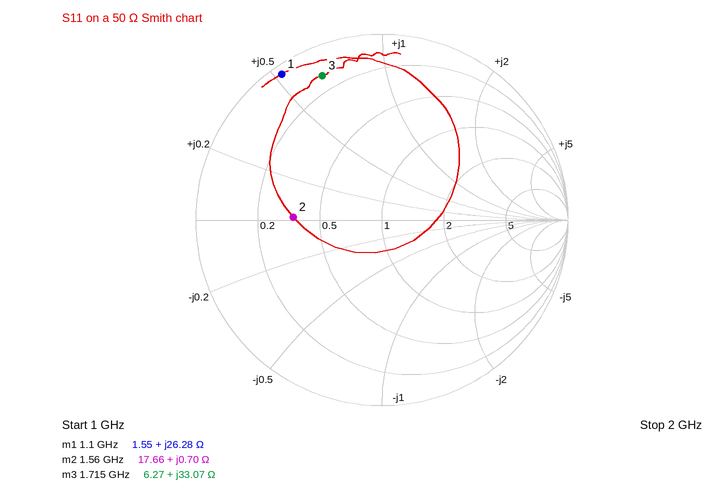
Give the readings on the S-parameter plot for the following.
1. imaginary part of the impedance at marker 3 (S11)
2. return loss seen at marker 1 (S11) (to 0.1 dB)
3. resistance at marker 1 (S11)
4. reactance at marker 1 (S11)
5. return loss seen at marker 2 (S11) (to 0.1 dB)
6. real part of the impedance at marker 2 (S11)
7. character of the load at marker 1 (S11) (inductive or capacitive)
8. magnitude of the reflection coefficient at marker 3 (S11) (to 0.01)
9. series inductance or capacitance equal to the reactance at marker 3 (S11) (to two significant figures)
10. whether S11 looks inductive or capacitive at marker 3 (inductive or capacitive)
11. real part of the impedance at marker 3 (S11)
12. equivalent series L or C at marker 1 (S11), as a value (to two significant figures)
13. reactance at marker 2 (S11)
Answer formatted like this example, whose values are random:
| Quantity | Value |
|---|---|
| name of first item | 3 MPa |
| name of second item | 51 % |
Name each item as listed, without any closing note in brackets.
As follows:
| Quantity | Value |
|---|---|
| imaginary part of the impedance at marker 3 | +33.07 Ω |
| return loss seen at marker 1 (S11) | 0.4 dB |
| resistance at marker 1 | 1.55 Ω |
| reactance at marker 1 | +26.28 Ω |
| return loss seen at marker 2 (S11) | 6.4 dB |
| real part of the impedance at marker 2 | 17.66 Ω |
| character of the load at marker 1 (S11) | inductive |
| magnitude of the reflection coefficient at marker 3 (S11) | 0.84 |
| series inductance or capacitance equal to the reactance at marker 3 (S11) | 3.1 nH |
| whether S11 looks inductive or capacitive at marker 3 | inductive |
| real part of the impedance at marker 3 | 6.27 Ω |
| equivalent series L or C at marker 1 (S11), as a value | 3.8 nH |
| reactance at marker 2 | +0.70 Ω |
